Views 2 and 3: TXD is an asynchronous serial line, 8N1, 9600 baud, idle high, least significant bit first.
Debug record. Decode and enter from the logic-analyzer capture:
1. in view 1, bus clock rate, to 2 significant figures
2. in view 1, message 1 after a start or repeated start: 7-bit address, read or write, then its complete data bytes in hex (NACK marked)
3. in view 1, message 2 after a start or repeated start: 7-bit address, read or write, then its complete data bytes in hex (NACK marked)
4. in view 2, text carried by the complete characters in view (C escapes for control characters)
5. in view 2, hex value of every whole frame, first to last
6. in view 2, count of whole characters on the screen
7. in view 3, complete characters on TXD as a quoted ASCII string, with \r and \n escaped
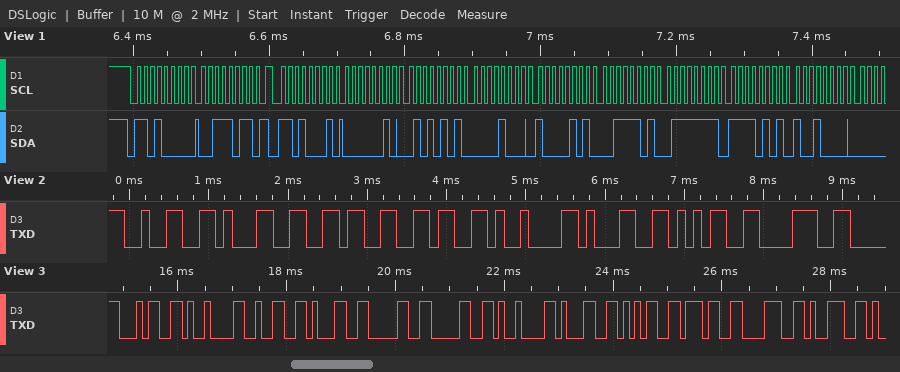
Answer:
100 kHz
0x68 write: 3B
0x68 read: 02 55 08 85 3D 7F F5 90
"2166\t158"
32 31 36 36 09 31 35 38
8
"4\t2100\t15789"
